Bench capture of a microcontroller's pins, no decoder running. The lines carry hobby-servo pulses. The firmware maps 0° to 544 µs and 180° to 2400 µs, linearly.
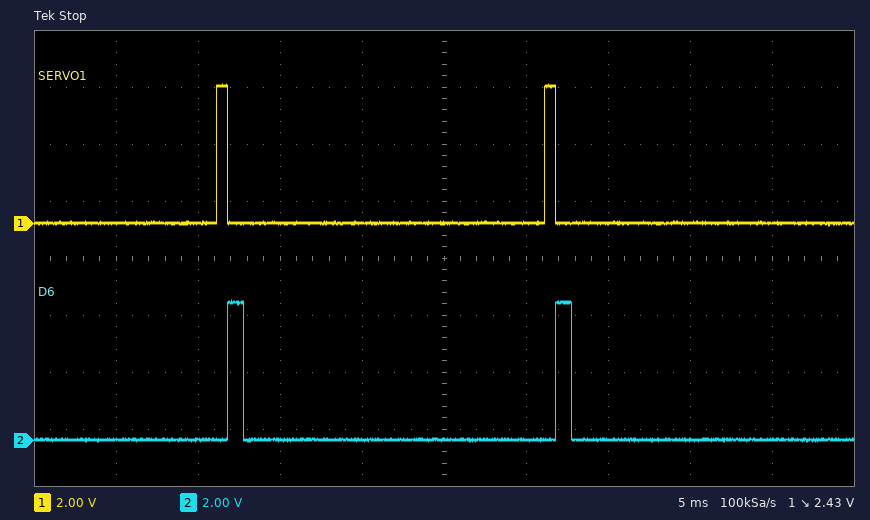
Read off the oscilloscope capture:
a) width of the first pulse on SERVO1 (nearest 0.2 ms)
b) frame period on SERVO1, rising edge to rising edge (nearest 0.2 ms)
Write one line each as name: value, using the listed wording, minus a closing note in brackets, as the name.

width of the first pulse on SERVO1: 0.6 ms
frame period on SERVO1, rising edge to rising edge: 20.0 ms
